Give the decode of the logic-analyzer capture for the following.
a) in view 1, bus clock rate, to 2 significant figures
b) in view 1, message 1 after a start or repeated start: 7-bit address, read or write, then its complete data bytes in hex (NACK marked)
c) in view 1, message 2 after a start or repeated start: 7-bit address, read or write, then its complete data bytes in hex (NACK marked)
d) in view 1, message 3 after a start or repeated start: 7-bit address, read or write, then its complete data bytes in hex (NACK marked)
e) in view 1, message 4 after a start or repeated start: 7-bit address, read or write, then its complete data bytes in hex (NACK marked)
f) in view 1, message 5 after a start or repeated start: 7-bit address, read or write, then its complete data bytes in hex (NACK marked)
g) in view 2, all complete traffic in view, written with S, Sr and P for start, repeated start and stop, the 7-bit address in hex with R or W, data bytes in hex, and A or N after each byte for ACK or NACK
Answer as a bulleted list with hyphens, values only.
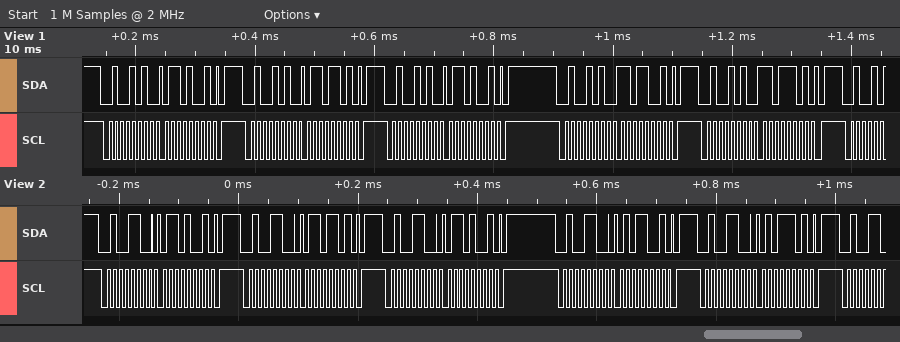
- 100 kHz
- 0x25 write: 69
- 0x25 write: 6D
- 0x25 write: 69
- 0x25 write: D9
- 0x25 write: DD
- S 26W A 69 A P S 26W A 6D A P S 26W A 69 A P S 26W A 59 A P S 26W A 5D A P
